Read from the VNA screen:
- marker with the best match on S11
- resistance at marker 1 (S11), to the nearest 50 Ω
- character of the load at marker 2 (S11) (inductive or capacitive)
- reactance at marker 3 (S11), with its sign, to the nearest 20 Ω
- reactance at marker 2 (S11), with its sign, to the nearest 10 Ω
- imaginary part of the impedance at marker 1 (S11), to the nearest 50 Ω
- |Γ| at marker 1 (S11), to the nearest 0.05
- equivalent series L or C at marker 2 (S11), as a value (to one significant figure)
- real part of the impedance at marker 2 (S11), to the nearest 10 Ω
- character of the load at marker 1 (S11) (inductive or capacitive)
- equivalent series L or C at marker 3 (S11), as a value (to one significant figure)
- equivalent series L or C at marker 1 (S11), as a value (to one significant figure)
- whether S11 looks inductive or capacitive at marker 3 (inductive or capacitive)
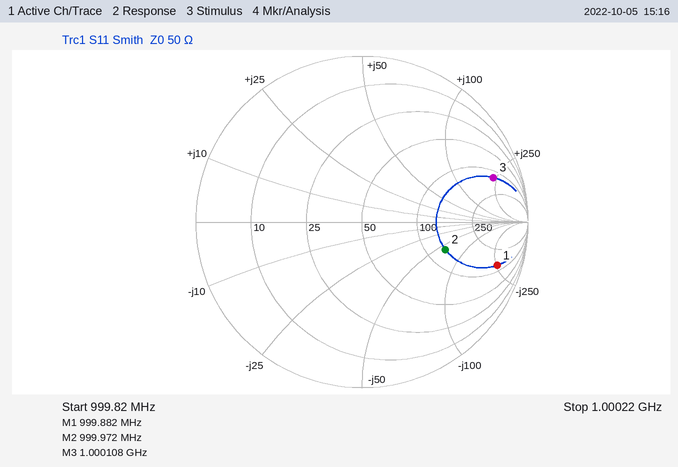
marker 2
150 Ω
capacitive
+240 Ω
-60 Ω
-250 Ω
0.85
3 pF
130 Ω
capacitive
40 nH
600 fF
inductive
